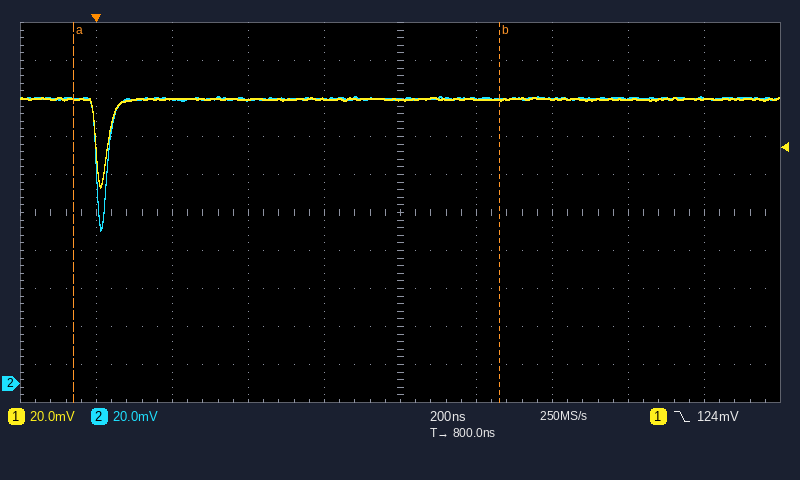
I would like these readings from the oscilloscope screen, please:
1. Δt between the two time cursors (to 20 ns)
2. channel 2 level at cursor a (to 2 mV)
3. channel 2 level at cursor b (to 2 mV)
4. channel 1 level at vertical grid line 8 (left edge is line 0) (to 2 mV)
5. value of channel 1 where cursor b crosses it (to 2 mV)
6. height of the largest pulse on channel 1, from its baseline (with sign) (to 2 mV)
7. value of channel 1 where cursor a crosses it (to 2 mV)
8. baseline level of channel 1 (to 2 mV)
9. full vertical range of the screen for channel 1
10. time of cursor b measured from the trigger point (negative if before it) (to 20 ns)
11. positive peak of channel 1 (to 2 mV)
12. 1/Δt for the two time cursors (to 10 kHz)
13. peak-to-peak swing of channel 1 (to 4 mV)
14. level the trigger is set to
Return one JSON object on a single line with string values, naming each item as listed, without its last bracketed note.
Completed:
{"Δt between the two time cursors": "1.12 µs", "channel 2 level at cursor a": "150 mV", "channel 2 level at cursor b": "150 mV", "channel 1 level at vertical grid line 8 (left edge is line 0)": "150 mV", "value of channel 1 where cursor b crosses it": "150 mV", "height of the largest pulse on channel 1, from its baseline (with sign)": "-46 mV", "value of channel 1 where cursor a crosses it": "150 mV", "baseline level of channel 1": "150 mV", "full vertical range of the screen for channel 1": "200 mV", "time of cursor b measured from the trigger point (negative if before it)": "+1.06 µs", "positive peak of channel 1": "150 mV", "1/Δt for the two time cursors": "890 kHz", "peak-to-peak swing of channel 1": "48 mV", "level the trigger is set to": "124 mV"}
